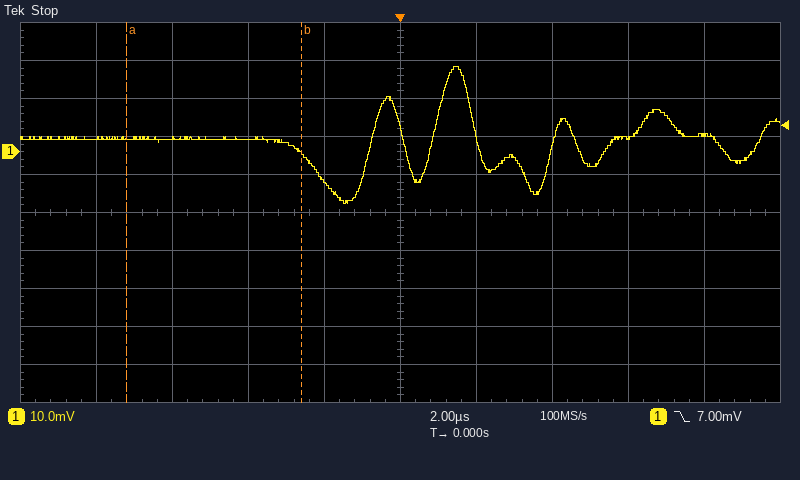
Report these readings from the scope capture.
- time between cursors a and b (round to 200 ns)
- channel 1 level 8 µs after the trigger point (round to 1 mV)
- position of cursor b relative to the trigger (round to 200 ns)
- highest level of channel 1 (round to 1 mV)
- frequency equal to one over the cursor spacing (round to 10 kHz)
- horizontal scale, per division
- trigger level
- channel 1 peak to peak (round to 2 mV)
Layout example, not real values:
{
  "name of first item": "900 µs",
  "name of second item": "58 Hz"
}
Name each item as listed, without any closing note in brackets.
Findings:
{
  "time between cursors a and b": "4.6 µs",
  "channel 1 level 8 µs after the trigger point": "4 mV",
  "position of cursor b relative to the trigger": "-2.6 µs",
  "highest level of channel 1": "22 mV",
  "frequency equal to one over the cursor spacing": "220 kHz",
  "horizontal scale, per division": "2 µs",
  "trigger level": "7.00 mV",
  "channel 1 peak to peak": "36 mV"
}
